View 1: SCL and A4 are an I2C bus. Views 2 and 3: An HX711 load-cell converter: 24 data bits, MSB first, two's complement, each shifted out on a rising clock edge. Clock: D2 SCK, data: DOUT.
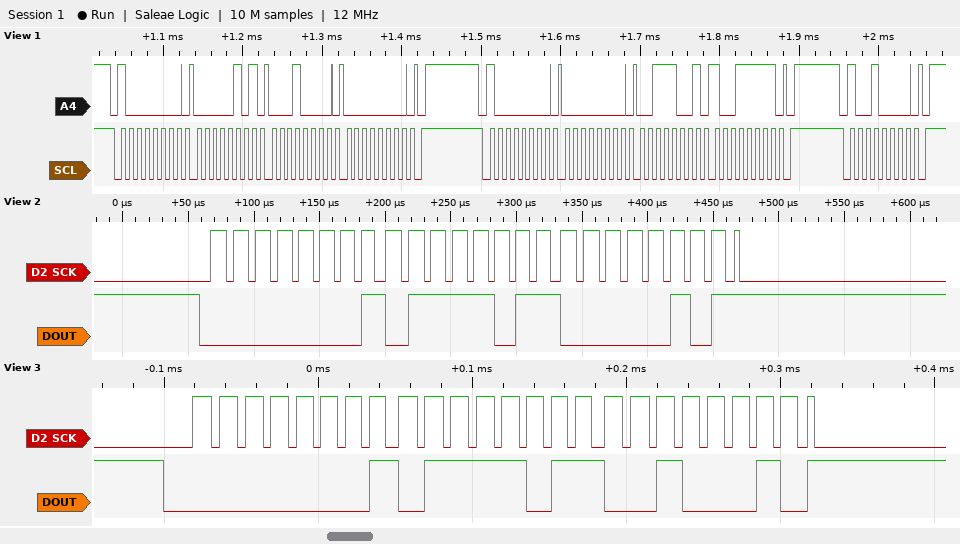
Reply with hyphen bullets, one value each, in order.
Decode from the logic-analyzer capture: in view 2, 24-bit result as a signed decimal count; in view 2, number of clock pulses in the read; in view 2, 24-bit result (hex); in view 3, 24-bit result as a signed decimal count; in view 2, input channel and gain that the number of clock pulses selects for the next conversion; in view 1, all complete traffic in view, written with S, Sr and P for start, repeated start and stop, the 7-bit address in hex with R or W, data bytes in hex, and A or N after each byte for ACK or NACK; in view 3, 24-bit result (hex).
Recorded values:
- 97029
- 25
- 0x017B05
- 97058
- channel A, gain 128
- S 40W A 05 A 10 A 00 A P S 40W A 00 A 39 A 9F A P S 48W A P
- 0x017B22
